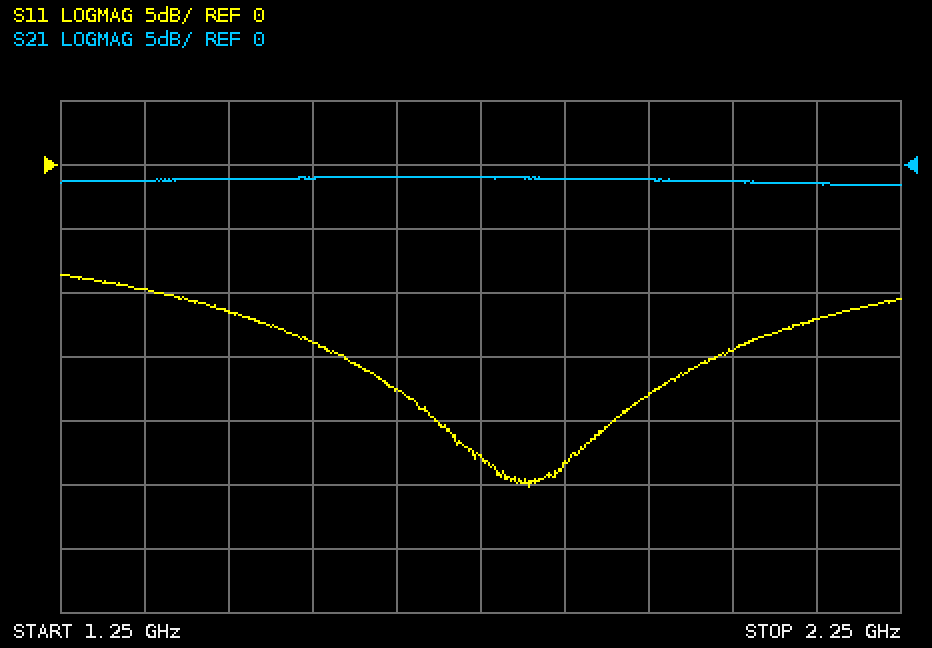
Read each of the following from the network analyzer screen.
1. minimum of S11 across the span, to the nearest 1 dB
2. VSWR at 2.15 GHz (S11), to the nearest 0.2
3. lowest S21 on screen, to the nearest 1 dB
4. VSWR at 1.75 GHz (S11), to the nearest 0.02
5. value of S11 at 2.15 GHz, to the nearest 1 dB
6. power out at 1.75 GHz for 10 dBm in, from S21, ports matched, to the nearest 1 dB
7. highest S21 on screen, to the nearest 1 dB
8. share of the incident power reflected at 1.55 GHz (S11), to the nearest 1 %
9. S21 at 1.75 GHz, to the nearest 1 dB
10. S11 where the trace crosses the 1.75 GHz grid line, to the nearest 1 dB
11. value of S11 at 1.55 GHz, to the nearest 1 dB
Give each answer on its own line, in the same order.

-25 dB
1.6
-2 dB
1.16
-12 dB
9 dBm
-1 dB
4 %
-1 dB
-23 dB
-14 dB
